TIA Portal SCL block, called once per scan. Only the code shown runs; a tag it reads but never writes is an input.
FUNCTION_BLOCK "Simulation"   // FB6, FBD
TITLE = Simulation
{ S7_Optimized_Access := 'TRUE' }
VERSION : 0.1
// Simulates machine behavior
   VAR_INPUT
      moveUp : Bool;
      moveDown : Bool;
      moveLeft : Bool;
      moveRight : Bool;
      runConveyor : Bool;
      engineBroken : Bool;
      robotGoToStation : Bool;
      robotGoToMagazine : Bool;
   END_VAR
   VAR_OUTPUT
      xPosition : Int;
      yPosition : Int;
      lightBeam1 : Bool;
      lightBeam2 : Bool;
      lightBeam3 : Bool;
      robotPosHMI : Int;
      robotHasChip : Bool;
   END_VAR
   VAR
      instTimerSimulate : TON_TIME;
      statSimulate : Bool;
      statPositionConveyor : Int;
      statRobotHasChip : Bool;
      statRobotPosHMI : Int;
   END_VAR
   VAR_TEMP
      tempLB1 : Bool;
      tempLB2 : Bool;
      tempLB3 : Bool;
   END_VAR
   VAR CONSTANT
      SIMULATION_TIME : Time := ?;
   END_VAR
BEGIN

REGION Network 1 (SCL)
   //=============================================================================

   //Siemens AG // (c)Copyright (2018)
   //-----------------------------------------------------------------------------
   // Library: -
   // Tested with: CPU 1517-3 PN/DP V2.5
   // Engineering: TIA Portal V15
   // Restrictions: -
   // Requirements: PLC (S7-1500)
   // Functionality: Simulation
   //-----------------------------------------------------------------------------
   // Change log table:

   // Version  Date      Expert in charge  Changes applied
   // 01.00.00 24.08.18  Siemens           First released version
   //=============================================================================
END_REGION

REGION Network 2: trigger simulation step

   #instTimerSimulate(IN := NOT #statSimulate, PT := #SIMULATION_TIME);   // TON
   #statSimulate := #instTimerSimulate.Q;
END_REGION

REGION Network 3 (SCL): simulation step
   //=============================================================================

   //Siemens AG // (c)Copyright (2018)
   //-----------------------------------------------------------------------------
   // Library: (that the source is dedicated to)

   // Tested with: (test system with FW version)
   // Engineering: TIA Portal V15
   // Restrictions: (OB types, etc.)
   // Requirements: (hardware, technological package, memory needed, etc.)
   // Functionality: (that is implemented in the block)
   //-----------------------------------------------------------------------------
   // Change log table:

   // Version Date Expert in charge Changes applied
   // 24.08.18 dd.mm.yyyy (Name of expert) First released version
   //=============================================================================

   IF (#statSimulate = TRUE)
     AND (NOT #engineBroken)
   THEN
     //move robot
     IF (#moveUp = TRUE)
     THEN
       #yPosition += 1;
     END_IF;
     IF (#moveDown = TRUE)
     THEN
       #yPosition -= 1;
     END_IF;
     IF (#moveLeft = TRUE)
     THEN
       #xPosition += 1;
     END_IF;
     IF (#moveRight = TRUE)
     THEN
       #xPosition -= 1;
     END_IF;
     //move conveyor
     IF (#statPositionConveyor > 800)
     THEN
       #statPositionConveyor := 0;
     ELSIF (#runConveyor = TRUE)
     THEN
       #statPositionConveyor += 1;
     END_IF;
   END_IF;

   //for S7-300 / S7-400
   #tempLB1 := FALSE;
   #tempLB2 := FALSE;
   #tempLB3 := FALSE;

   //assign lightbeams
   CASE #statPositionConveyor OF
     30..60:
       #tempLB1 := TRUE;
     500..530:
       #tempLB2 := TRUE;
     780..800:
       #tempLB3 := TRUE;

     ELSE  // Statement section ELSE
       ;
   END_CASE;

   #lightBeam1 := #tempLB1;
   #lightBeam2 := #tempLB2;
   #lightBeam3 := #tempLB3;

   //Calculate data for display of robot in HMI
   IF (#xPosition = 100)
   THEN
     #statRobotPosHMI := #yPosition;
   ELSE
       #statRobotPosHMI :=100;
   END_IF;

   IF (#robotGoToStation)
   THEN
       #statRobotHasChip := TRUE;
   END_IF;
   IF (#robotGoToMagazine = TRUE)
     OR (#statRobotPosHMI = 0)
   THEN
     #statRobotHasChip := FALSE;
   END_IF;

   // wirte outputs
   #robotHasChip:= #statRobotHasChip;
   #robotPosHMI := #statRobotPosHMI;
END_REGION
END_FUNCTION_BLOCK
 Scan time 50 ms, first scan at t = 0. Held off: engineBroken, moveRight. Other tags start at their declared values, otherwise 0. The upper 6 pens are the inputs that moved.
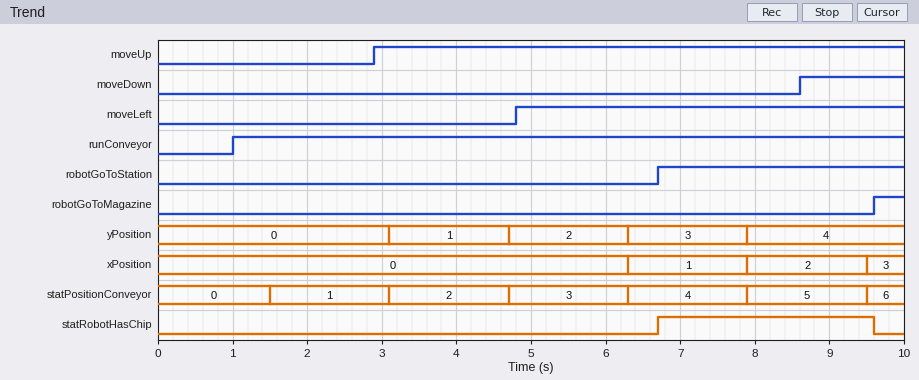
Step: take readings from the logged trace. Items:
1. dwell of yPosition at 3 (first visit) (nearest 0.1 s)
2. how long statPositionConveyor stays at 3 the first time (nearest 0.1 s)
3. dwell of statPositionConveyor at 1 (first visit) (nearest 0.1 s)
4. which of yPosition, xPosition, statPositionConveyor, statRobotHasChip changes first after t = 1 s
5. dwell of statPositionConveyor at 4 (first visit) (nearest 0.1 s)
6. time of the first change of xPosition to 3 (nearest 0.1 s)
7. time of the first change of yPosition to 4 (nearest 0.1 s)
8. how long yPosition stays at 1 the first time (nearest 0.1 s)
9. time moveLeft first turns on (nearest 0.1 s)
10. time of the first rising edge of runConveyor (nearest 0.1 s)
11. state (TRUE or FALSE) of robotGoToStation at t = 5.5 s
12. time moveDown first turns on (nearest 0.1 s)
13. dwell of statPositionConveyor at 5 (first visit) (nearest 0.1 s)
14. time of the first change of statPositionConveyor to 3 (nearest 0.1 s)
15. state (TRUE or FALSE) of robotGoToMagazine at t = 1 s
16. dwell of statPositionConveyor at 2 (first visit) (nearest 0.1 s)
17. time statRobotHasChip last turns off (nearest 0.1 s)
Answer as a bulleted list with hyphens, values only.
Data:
- 1.6 s
- 1.6 s
- 1.6 s
- statPositionConveyor
- 1.6 s
- 9.5 s
- 7.9 s
- 1.6 s
- 4.8 s
- 1.0 s
- FALSE
- 8.6 s
- 1.6 s
- 4.7 s
- FALSE
- 1.6 s
- 9.6 s
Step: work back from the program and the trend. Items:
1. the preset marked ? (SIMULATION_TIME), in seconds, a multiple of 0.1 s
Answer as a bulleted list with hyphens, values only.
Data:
- 1.5 s
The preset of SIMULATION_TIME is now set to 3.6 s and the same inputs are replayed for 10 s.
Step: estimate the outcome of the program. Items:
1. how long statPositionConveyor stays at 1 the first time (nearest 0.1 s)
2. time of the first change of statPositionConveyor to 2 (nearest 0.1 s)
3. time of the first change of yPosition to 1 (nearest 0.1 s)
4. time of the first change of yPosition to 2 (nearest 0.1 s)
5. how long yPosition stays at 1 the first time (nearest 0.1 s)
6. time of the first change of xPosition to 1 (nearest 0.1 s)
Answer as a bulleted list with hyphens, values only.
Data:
- 3.7 s
- 7.3 s
- 3.6 s
- 7.3 s
- 3.7 s
- 7.3 s
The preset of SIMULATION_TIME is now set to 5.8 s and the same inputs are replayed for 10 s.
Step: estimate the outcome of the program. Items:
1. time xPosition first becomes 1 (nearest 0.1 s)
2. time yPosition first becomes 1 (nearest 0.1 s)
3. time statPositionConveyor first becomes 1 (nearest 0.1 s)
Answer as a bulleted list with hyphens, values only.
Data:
- 5.8 s
- 5.8 s
- 5.8 s
